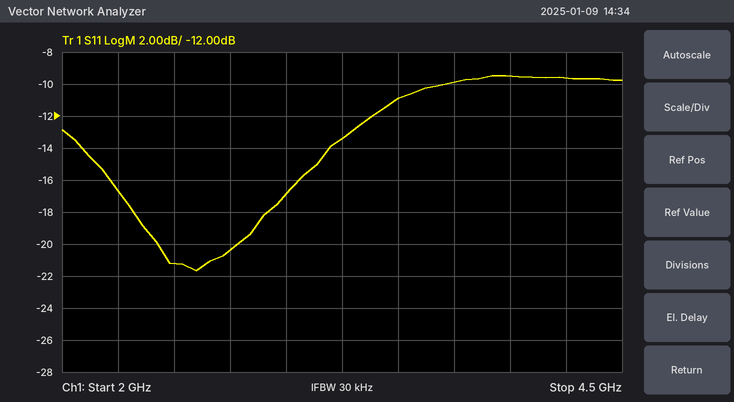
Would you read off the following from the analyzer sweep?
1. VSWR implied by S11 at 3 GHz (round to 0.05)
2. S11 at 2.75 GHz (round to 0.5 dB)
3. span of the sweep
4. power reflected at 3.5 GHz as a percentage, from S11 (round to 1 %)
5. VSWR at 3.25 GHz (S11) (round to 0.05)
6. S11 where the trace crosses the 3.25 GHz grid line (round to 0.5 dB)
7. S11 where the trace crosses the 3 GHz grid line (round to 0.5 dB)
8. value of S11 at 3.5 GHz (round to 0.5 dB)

1.35
-20.5 dB
2.5 GHz
8 %
1.55
-13.5 dB
-17.0 dB
-11.0 dB
